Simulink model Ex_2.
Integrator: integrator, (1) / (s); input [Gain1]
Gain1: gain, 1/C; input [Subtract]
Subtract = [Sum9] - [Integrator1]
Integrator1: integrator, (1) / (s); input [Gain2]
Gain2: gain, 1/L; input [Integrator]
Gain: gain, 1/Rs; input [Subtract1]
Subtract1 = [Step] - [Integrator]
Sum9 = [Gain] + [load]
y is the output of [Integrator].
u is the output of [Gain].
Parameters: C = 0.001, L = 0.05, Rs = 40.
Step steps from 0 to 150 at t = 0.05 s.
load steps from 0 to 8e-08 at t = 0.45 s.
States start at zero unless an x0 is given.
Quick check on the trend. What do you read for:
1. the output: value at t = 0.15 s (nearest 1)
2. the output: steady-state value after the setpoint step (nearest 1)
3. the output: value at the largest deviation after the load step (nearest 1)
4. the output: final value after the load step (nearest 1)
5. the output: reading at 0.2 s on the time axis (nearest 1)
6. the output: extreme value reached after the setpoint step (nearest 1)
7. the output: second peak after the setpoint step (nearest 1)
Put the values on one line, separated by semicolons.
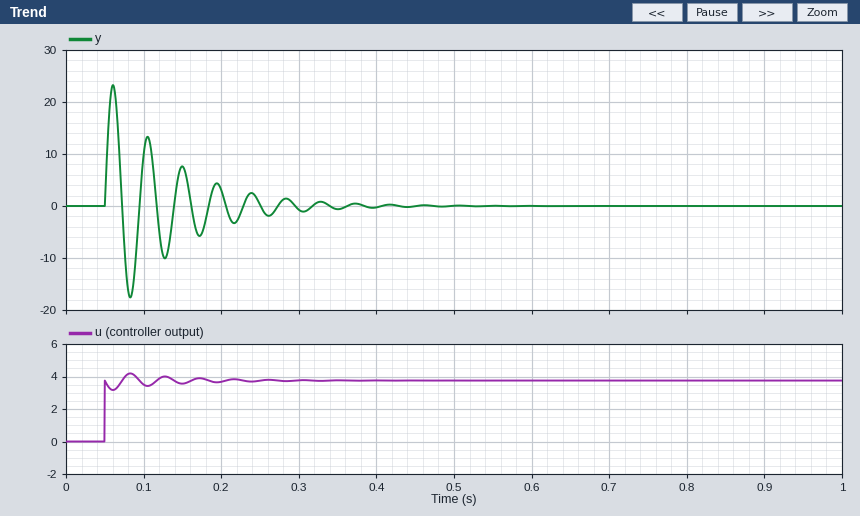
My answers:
8; 0; 0; 0; 3; 23; 13
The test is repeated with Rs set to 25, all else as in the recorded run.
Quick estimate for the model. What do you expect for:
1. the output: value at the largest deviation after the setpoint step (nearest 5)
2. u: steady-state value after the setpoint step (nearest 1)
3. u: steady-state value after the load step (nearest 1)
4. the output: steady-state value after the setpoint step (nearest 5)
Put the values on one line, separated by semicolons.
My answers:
35; 6; 6; 0
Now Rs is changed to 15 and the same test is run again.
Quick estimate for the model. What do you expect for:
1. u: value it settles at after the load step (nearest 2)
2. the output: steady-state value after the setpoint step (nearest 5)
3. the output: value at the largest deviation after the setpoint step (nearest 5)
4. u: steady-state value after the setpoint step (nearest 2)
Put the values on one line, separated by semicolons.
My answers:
10; 0; 50; 10
